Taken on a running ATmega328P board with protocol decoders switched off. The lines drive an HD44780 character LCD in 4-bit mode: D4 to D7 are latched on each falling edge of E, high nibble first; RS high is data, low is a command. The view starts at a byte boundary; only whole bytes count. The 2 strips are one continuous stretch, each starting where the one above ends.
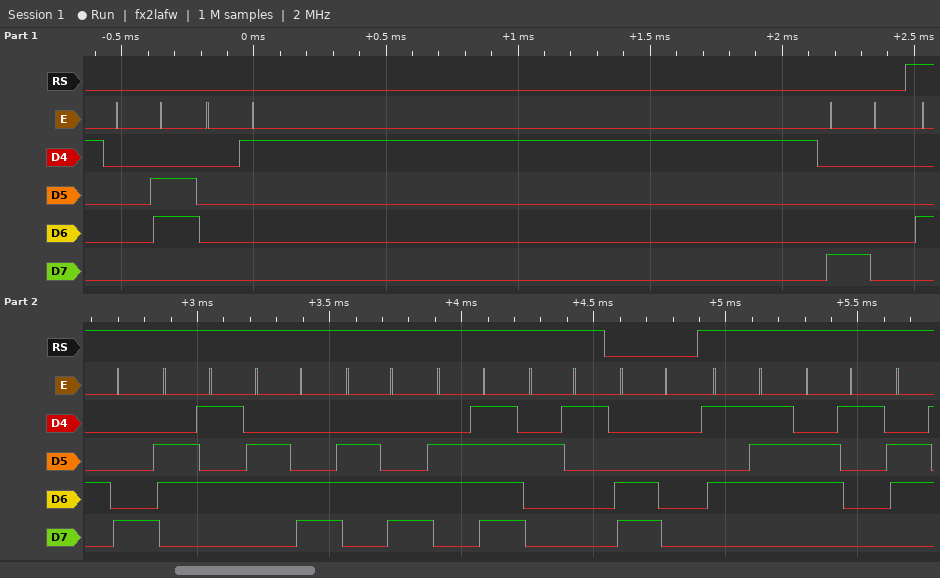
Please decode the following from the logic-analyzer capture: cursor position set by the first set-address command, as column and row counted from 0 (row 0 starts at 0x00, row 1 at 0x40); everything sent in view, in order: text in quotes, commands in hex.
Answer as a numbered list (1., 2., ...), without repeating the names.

1. column 0, row 0
2. 0x06 0x01 0x80 "Hello!" 0xC0 "Wa"
